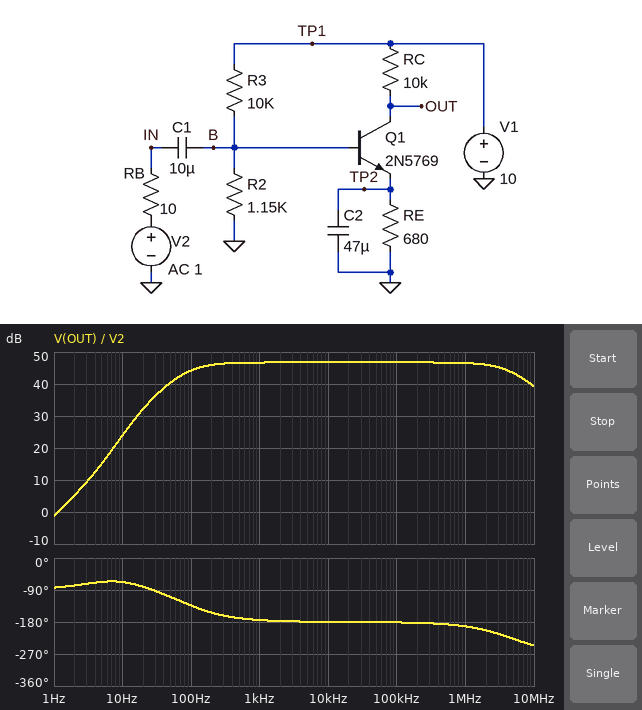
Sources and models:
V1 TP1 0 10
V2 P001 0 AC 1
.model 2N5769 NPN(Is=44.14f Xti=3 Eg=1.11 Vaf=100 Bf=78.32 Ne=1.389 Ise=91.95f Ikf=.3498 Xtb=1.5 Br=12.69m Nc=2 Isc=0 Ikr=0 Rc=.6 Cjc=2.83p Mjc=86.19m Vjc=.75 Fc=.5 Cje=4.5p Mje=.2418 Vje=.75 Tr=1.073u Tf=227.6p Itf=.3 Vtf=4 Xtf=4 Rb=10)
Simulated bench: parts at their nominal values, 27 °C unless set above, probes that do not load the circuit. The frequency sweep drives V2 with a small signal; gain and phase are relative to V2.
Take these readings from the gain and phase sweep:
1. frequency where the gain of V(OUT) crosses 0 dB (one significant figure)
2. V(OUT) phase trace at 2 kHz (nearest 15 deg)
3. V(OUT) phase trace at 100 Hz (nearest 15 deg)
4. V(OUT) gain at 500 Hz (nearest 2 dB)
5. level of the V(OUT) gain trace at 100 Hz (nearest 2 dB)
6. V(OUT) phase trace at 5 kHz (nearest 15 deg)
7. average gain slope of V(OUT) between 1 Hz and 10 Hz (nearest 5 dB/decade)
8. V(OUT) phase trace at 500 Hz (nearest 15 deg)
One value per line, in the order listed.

1 Hz
-180 deg
-135 deg
46 dB
44 dB
-180 deg
25 dB/decade
-165 deg
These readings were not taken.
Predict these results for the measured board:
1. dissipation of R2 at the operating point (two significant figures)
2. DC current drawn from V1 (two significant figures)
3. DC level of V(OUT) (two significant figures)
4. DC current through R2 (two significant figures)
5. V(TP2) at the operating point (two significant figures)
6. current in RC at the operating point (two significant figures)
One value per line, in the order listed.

910 µW
1.5 mA
3.9 V
890 µA
420 mV
610 µA
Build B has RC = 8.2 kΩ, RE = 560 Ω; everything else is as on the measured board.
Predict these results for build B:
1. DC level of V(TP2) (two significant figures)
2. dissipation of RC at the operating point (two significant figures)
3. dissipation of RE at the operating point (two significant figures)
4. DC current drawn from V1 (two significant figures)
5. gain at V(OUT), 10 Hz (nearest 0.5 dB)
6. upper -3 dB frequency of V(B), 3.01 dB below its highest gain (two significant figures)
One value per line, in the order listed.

410 mV
4.3 mW
300 µW
1.6 mA
22.5 dB
850 MHz
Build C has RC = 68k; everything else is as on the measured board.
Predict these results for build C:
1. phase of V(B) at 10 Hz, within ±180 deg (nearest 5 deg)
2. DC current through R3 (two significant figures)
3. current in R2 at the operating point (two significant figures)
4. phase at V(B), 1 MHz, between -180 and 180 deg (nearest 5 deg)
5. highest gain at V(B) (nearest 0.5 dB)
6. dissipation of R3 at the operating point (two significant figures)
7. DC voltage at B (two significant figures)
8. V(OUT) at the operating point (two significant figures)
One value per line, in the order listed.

45 deg
920 µA
720 µA
0 deg
-1.0 dB
8.4 mW
820 mV
360 mV
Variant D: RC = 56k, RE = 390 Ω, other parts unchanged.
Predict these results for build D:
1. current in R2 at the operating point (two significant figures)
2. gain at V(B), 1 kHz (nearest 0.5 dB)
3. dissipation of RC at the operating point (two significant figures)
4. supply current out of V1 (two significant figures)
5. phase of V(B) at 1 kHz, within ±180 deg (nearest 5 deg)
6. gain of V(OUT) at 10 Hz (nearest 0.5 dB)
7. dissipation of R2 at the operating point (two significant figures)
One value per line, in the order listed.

670 µA
-1.5 dB
1.7 mW
1.1 mA
10 deg
-19.5 dB
510 µW
